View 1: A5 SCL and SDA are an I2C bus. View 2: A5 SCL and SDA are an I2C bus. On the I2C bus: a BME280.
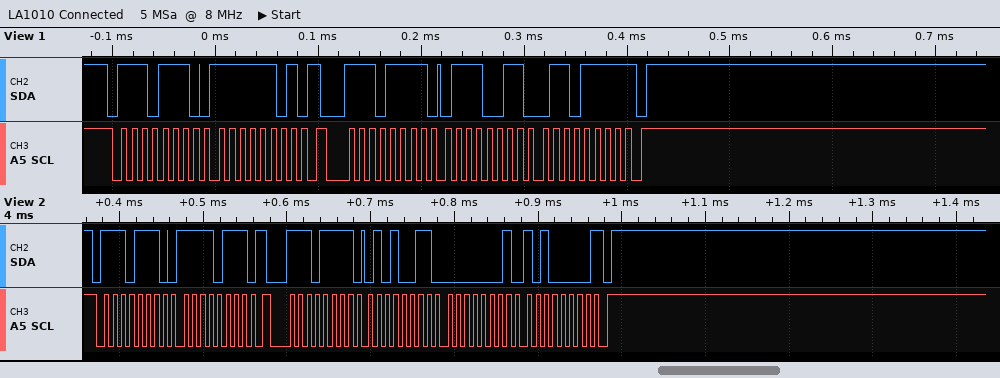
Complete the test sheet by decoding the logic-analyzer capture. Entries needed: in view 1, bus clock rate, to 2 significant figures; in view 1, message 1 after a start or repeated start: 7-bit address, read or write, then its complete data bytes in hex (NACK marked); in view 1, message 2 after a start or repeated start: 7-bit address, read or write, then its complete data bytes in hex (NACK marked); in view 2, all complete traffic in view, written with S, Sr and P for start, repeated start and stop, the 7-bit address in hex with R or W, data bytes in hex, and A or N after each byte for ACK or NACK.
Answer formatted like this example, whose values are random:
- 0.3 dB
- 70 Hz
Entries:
- 100 kHz
- 0x77 write: FD
- 0x77 read: 73 6F NACK
- S 77W A F7 A Sr 77R A 53 A 01 A A0 N P
